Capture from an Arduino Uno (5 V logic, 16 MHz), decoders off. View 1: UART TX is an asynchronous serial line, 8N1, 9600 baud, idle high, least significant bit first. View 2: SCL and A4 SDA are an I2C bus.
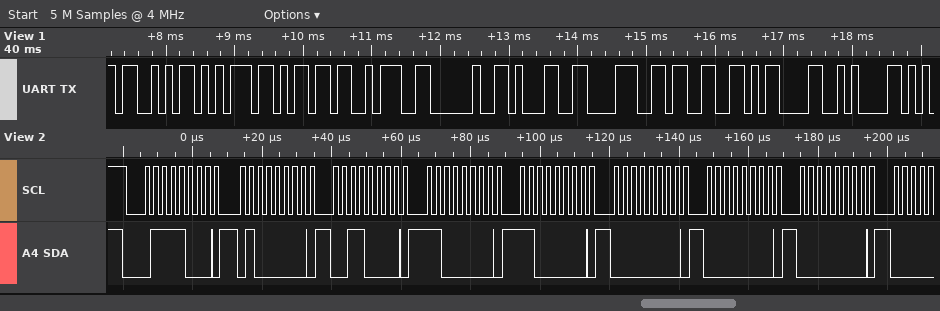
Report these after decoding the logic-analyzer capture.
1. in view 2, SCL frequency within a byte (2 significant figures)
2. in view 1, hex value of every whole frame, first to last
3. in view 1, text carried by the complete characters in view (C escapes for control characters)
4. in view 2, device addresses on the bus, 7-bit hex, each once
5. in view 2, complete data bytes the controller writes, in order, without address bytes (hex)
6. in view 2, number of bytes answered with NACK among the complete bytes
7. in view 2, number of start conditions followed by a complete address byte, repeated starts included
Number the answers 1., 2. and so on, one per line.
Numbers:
1. 400 kHz
2. 53 75 6D 3A 20 31 38 33 0D 0A
3. "Sum: 183\r\n"
4. 0x3C
5. 40 30 C0 C0 00 00 00
6. 0
7. 1
